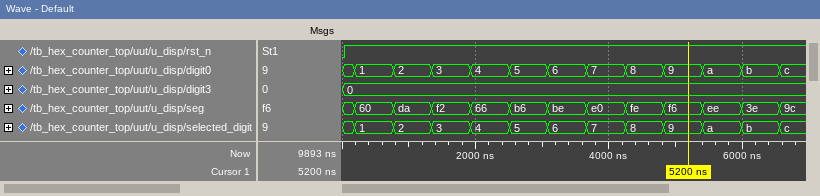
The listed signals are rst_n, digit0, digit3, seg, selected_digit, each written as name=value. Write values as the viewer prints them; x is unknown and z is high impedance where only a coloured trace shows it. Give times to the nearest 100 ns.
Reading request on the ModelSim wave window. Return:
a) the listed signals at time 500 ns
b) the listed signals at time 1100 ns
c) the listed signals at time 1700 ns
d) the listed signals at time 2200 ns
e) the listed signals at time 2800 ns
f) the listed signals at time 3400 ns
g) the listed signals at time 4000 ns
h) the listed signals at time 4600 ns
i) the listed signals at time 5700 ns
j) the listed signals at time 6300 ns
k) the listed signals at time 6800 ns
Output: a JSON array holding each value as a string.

["rst_n=1, digit0=1, digit3=0, seg=60, selected_digit=1", "rst_n=1, digit0=2, digit3=0, seg=da, selected_digit=2", "rst_n=1, digit0=3, digit3=0, seg=f2, selected_digit=3", "rst_n=1, digit0=4, digit3=0, seg=66, selected_digit=4", "rst_n=1, digit0=5, digit3=0, seg=b6, selected_digit=5", "rst_n=1, digit0=6, digit3=0, seg=be, selected_digit=6", "rst_n=1, digit0=7, digit3=0, seg=e0, selected_digit=7", "rst_n=1, digit0=8, digit3=0, seg=fe, selected_digit=8", "rst_n=1, digit0=a, digit3=0, seg=ee, selected_digit=a", "rst_n=1, digit0=b, digit3=0, seg=3e, selected_digit=b", "rst_n=1, digit0=c, digit3=0, seg=9c, selected_digit=c"]
